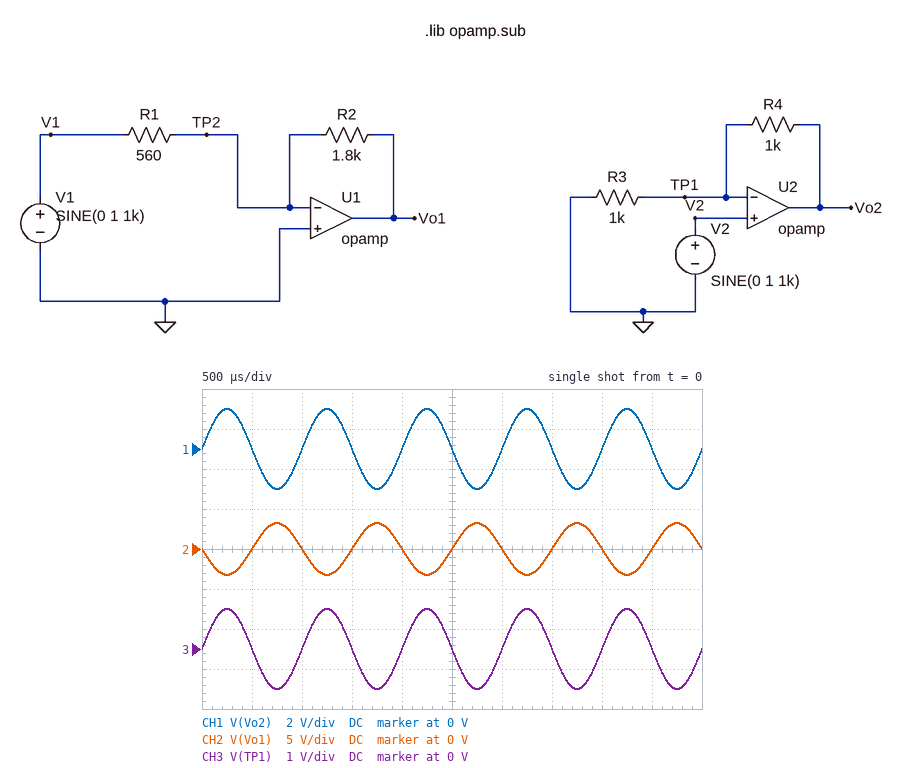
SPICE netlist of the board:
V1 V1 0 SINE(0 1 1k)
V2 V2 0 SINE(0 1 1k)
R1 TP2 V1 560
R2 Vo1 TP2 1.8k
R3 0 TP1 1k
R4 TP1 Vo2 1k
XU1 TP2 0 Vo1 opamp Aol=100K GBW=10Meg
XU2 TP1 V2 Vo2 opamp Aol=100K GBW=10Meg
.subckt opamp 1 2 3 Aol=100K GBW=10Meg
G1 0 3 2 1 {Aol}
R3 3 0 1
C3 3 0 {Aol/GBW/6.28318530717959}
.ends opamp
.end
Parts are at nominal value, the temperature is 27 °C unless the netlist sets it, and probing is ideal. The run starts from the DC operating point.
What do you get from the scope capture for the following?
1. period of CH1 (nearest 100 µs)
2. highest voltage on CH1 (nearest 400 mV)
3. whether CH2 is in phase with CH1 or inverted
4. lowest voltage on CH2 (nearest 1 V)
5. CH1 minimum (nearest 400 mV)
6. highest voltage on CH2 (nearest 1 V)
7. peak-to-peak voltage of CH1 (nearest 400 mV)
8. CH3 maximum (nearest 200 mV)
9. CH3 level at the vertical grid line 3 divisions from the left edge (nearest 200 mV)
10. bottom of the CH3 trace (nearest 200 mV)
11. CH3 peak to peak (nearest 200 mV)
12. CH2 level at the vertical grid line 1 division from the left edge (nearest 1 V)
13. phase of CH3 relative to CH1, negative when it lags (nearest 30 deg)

1.0 ms
2.0 V
inverted
-3 V
-2.0 V
3 V
4.0 V
1.0 V
0 V
-1.0 V
2.0 V
0 V
0 deg
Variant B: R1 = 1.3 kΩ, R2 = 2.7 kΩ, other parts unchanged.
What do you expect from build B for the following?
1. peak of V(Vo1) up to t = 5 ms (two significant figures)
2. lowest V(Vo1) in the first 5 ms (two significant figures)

2.1 V
-2.1 V
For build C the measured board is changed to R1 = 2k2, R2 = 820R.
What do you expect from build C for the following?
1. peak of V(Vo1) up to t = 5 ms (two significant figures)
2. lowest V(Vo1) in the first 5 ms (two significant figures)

370 mV
-370 mV
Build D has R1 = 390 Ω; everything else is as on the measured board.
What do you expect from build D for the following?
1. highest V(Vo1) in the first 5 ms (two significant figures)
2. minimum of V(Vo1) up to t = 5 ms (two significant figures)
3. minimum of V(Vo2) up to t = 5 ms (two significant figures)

4.6 V
-4.6 V
-2.0 V
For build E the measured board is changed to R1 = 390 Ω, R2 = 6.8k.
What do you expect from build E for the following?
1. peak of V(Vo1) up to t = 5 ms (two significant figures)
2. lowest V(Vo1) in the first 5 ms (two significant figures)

17 V
-17 V
